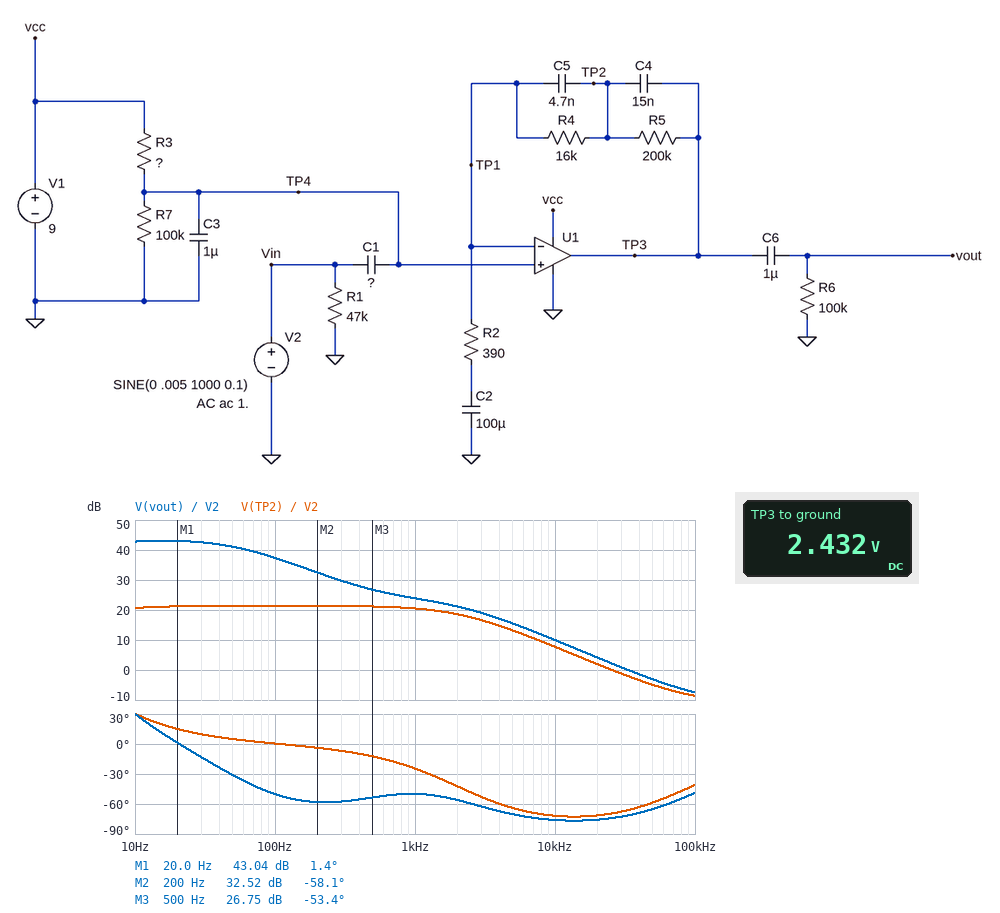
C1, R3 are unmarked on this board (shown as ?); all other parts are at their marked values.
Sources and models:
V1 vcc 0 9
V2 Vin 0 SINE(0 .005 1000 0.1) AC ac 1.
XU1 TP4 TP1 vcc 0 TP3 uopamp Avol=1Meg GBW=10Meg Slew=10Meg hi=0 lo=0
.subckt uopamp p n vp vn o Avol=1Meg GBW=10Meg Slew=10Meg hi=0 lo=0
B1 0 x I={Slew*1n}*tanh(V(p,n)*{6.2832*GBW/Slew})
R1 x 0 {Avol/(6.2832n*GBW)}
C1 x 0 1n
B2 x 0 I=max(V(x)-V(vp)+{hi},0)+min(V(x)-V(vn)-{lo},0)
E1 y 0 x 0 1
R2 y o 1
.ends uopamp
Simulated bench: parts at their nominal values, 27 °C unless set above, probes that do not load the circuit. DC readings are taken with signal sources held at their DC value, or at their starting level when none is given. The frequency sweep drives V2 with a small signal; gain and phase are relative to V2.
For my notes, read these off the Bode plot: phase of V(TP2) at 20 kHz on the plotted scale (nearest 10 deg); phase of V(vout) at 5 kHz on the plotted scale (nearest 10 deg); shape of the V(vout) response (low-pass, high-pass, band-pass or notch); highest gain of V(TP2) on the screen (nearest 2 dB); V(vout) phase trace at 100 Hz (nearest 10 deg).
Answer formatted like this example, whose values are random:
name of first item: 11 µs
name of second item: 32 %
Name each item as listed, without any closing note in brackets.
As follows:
phase of V(TP2) at 20 kHz on the plotted scale: -70 deg
phase of V(vout) at 5 kHz on the plotted scale: -70 deg
shape of the V(vout) response: low-pass
highest gain of V(TP2) on the screen: 22 dB
V(vout) phase trace at 100 Hz: -50 deg
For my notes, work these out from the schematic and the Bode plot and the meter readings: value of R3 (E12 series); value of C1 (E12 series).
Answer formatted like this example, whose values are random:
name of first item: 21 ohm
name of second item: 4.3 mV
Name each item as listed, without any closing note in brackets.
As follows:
value of R3: 270 kΩ
value of C1: 390 nF
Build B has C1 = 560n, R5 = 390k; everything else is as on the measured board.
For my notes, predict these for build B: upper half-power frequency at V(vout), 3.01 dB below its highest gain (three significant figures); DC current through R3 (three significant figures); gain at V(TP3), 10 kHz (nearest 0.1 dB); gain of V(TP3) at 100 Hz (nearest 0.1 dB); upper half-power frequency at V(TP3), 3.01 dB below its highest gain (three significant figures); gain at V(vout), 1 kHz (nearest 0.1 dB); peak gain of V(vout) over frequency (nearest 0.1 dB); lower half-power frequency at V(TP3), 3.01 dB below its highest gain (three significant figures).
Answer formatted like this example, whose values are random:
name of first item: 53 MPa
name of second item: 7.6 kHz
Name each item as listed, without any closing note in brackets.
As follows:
upper half-power frequency at V(vout), 3.01 dB below its highest gain: 35.5 Hz
DC current through R3: 24.3 µA
gain at V(TP3), 10 kHz: 12.1 dB
gain of V(TP3) at 100 Hz: 40.0 dB
upper half-power frequency at V(TP3), 3.01 dB below its highest gain: 35.0 Hz
gain at V(vout), 1 kHz: 26.0 dB
peak gain of V(vout) over frequency: 50.1 dB
lower half-power frequency at V(TP3), 3.01 dB below its highest gain: 3.58 Hz
